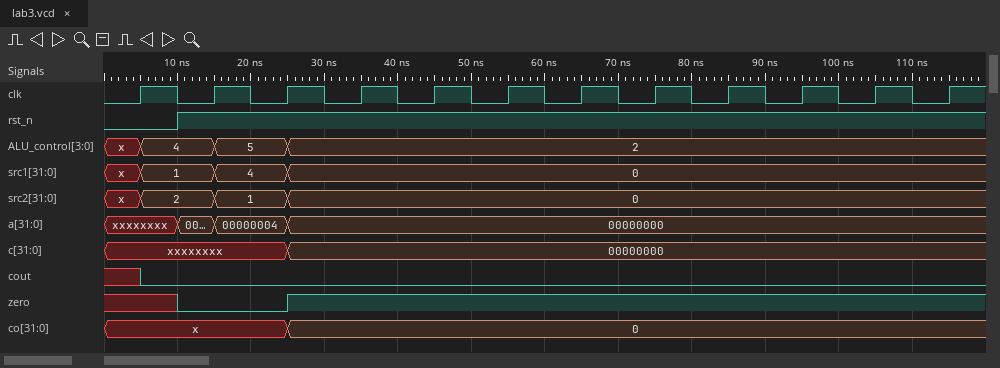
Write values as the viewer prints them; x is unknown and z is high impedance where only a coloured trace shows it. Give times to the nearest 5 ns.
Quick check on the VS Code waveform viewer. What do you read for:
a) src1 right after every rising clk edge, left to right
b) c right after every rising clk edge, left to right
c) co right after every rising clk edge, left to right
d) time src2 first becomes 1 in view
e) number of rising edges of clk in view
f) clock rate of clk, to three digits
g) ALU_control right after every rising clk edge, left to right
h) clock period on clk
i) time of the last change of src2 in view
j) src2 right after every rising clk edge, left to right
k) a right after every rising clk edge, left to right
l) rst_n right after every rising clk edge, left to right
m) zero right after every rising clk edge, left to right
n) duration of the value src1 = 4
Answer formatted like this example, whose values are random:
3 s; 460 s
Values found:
1, 4, 0, 0, 0, 0, 0, 0, 0, 0, 0, 0; xxxxxxxx, xxxxxxxx, 00000000, 00000000, 00000000, 00000000, 00000000, 00000000, 00000000, 00000000, 00000000, 00000000; x, x, 0, 0, 0, 0, 0, 0, 0, 0, 0, 0; 15 ns; 12; 100 MHz; 4, 5, 2, 2, 2, 2, 2, 2, 2, 2, 2, 2; 10 ns; 25 ns; 2, 1, 0, 0, 0, 0, 0, 0, 0, 0, 0, 0; xxxxxxxx, 00000004, 00000000, 00000000, 00000000, 00000000, 00000000, 00000000, 00000000, 00000000, 00000000, 00000000; 0 1 1 1 1 1 1 1 1 1 1 1; x 0 1 1 1 1 1 1 1 1 1 1; 10 ns
